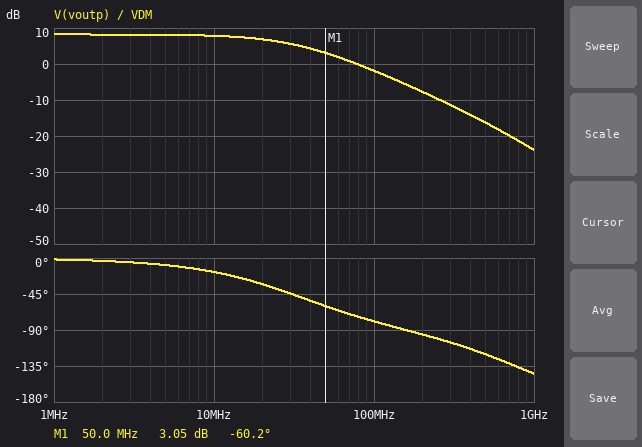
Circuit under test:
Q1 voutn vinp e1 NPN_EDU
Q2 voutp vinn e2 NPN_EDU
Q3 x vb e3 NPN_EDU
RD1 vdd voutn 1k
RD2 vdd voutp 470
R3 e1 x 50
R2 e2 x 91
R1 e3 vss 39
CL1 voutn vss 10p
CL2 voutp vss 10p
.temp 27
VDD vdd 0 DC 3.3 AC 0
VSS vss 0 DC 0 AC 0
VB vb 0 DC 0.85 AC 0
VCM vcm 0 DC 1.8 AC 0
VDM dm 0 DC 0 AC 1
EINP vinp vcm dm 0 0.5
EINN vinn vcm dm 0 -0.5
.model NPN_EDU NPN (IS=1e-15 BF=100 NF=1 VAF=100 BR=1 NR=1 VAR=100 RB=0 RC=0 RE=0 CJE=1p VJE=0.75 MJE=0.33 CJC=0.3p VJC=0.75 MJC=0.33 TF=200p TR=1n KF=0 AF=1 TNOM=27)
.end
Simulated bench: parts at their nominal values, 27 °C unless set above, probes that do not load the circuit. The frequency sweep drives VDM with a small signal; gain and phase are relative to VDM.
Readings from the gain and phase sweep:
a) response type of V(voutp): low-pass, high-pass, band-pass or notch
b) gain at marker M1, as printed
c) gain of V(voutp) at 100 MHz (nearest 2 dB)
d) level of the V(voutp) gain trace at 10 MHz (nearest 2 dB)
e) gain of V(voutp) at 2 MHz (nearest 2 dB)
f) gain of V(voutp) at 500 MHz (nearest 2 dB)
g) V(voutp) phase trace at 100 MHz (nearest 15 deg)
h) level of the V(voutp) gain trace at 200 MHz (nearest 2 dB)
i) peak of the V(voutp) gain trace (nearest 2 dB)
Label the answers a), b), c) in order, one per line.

a) low-pass
b) 3.05 dB
c) -2 dB
d) 8 dB
e) 8 dB
f) -16 dB
g) -75 deg
h) -8 dB
i) 8 dB
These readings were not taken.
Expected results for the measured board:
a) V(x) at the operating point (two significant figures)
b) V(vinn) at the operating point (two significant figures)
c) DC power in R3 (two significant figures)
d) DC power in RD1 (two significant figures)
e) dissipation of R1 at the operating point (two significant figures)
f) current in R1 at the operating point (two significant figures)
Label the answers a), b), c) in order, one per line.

a) 990 mV
b) 1.8 V
c) 140 µW
d) 2.8 mW
e) 300 µW
f) 2.8 mA
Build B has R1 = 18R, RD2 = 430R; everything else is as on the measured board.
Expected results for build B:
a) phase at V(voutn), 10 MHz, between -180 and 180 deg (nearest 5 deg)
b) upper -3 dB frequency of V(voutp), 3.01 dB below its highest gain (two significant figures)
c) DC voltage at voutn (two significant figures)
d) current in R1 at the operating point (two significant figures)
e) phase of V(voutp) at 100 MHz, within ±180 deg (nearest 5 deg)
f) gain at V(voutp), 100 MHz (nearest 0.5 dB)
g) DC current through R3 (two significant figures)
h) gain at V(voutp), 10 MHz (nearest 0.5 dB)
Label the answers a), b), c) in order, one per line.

a) 0 deg
b) 36 MHz
c) 1.1 V
d) 5.2 mA
e) -75 deg
f) -1.0 dB
g) 3.2 mA
h) 8.0 dB
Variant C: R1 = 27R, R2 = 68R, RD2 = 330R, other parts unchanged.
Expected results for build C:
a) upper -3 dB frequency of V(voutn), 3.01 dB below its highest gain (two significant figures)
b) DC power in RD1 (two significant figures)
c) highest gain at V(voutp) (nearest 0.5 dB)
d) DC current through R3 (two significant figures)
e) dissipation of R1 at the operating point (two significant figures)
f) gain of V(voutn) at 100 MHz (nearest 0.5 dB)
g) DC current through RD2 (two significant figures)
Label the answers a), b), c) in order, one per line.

a) 17 MHz
b) 4.2 mW
c) 7.0 dB
d) 2.1 mA
e) 380 µW
f) 0 dB
g) 1.6 mA
